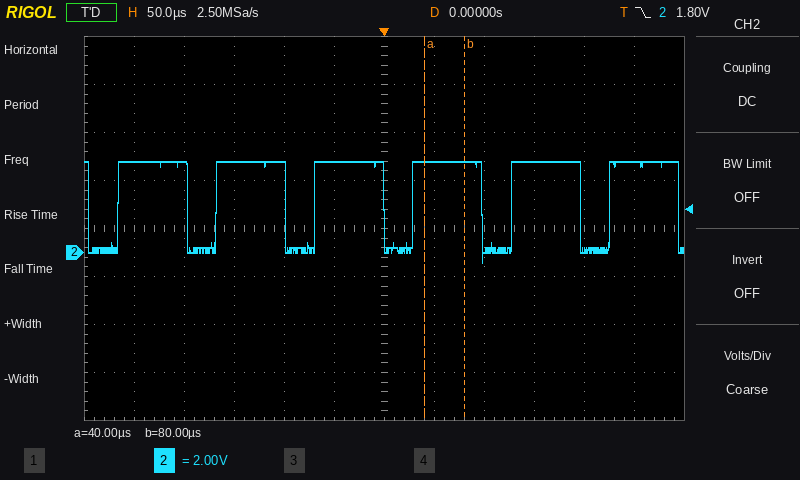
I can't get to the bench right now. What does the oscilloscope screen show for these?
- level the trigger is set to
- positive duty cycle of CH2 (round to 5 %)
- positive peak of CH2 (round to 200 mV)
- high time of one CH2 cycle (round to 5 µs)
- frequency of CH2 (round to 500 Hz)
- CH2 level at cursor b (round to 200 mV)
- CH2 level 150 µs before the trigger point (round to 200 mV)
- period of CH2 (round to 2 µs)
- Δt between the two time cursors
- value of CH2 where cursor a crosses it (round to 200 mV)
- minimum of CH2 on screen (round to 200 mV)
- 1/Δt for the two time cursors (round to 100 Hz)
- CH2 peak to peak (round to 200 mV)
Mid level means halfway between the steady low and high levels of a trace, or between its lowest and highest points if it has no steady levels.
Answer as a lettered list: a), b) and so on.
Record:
a) 1.80 V
b) 70 %
c) 3.8 V
d) 70 µs
e) 10.0 kHz
f) 3.8 V
g) 3.8 V
h) 98 µs
i) 40 µs
j) 3.8 V
k) -400 mV
l) 25.0 kHz
m) 4.2 V
